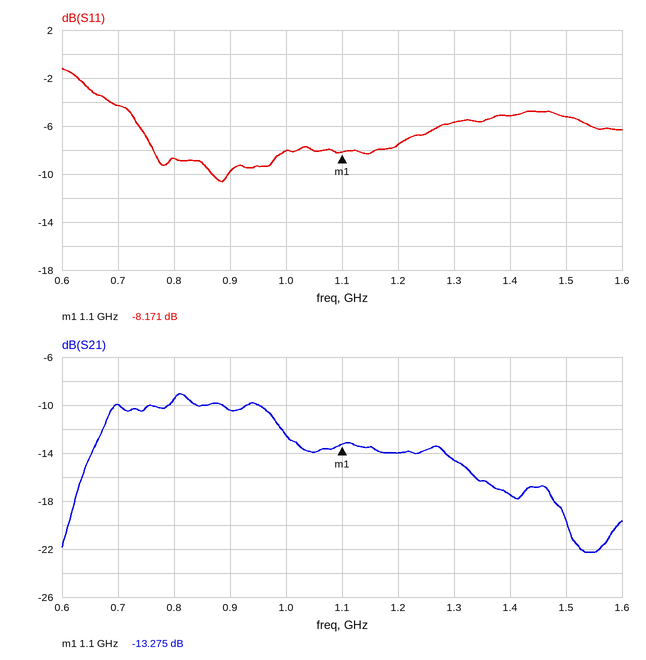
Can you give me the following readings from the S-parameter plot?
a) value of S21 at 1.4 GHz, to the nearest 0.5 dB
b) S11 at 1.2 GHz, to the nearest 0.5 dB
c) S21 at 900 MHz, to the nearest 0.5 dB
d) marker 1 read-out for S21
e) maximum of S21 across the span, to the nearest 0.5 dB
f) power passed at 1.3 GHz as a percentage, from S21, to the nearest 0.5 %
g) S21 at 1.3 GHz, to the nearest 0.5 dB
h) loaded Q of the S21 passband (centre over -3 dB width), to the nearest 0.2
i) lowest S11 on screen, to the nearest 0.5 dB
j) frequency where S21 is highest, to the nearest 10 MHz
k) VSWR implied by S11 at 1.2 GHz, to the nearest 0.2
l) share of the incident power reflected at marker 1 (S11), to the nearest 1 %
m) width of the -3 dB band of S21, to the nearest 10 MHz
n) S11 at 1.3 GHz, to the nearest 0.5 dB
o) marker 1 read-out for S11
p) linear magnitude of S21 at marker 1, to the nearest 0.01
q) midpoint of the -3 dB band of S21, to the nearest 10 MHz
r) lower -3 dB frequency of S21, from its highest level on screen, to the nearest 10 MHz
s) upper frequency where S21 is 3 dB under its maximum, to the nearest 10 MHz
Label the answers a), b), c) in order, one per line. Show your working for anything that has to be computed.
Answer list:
a) -17.5 dB
b) -7.5 dB
c) -10.5 dB
d) -13.275 dB
e) -9.0 dB
f) 10^(-14.5/10) ≈ 3.5 %
g) -14.5 dB
h) 830 MHz / 320 MHz ≈ 2.6
i) -10.5 dB
j) 810 MHz
k) |Γ| = 10^(-7.5/20) = 0.4217; VSWR = (1 + 0.4217)/(1 − 0.4217) ≈ 2.46, so 2.4 to the nearest 0.2
l) 10^(-8.171/10) ≈ 15 %
m) 990 MHz − 670 MHz = 320 MHz
n) -5.5 dB
o) -8.171 dB
p) 10^(-13.275/20) ≈ 0.22
q) 830 MHz
r) 670 MHz
s) 990 MHz
